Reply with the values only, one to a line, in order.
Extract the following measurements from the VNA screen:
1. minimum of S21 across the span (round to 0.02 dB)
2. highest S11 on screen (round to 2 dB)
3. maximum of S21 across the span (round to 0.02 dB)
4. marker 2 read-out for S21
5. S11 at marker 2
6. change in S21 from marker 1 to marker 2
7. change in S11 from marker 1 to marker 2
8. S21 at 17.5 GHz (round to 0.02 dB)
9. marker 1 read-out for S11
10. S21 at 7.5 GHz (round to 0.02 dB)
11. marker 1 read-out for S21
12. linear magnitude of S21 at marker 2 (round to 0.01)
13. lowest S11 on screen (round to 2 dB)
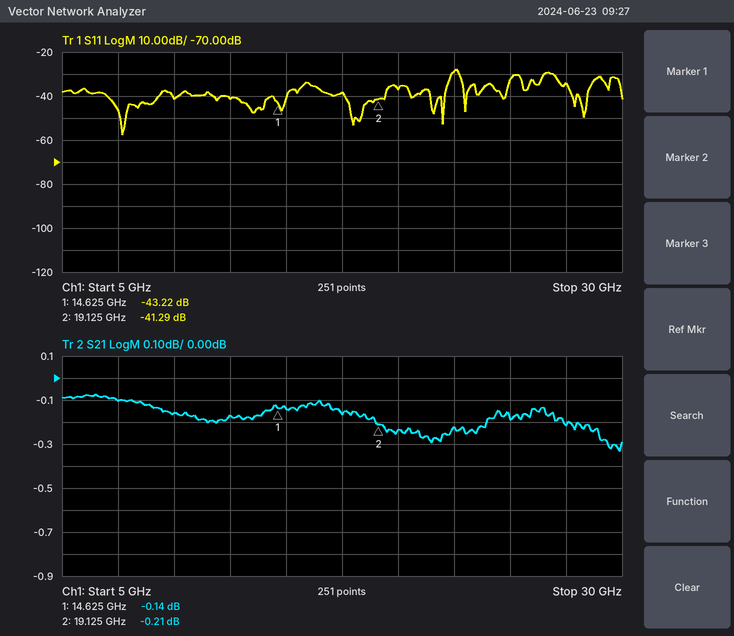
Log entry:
-0.34 dB
-28 dB
-0.08 dB
-0.21 dB
-41.29 dB
-0.07 dB
1.93 dB
-0.16 dB
-43.22 dB
-0.10 dB
-0.14 dB
0.98
-58 dB
